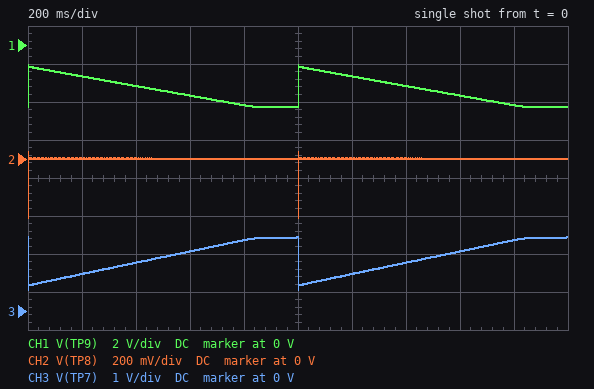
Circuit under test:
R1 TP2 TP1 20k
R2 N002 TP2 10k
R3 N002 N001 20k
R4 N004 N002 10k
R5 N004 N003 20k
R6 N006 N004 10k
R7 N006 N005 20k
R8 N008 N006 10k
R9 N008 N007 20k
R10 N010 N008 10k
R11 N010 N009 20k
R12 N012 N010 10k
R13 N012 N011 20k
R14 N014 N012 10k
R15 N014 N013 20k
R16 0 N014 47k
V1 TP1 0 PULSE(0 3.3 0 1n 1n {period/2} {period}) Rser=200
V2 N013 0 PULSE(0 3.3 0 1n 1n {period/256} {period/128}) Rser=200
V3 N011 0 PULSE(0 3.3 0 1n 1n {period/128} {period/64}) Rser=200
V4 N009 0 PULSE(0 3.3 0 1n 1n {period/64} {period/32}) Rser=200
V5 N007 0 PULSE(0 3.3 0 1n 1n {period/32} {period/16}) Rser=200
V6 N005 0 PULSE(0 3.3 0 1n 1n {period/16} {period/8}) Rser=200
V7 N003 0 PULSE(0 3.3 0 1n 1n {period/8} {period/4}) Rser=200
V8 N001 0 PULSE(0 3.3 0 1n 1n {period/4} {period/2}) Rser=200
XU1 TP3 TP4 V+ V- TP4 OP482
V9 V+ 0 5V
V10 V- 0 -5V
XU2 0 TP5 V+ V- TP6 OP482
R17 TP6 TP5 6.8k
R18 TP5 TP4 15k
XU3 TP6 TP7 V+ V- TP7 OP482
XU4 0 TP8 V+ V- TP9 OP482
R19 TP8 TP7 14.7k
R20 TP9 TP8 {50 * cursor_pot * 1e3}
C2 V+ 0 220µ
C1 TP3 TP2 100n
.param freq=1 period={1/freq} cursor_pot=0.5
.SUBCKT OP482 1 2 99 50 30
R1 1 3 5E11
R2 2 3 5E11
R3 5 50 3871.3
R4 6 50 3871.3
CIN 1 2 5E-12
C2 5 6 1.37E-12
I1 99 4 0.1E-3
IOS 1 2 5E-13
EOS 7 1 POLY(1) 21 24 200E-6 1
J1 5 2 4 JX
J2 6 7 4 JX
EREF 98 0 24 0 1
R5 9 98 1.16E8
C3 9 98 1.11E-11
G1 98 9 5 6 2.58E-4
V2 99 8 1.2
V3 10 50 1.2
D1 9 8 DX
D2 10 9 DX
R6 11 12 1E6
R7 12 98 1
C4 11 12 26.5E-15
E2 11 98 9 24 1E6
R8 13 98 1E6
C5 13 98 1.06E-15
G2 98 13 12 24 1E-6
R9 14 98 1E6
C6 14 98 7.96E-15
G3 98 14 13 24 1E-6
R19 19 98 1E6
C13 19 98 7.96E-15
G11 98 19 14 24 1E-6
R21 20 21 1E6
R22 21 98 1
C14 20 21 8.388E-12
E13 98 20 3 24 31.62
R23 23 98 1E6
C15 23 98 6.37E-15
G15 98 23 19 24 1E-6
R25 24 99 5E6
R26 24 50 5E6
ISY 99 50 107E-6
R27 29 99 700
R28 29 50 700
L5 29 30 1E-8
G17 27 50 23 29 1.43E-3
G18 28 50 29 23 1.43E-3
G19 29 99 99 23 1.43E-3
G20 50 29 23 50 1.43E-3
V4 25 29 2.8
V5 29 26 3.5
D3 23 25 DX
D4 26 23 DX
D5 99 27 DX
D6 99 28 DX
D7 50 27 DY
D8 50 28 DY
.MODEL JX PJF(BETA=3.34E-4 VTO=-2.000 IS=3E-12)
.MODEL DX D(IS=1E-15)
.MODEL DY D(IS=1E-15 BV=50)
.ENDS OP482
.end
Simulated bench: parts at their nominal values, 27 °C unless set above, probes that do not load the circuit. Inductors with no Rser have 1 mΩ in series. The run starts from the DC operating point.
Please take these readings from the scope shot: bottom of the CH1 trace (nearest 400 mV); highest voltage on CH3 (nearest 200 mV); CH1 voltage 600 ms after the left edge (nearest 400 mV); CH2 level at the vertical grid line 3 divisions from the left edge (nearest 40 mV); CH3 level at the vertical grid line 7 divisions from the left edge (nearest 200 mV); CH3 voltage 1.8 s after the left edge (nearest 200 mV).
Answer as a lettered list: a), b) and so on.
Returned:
a) -3.2 V
b) 2.0 V
c) -2.8 V
d) 0 V
e) 1.2 V
f) 1.8 V
